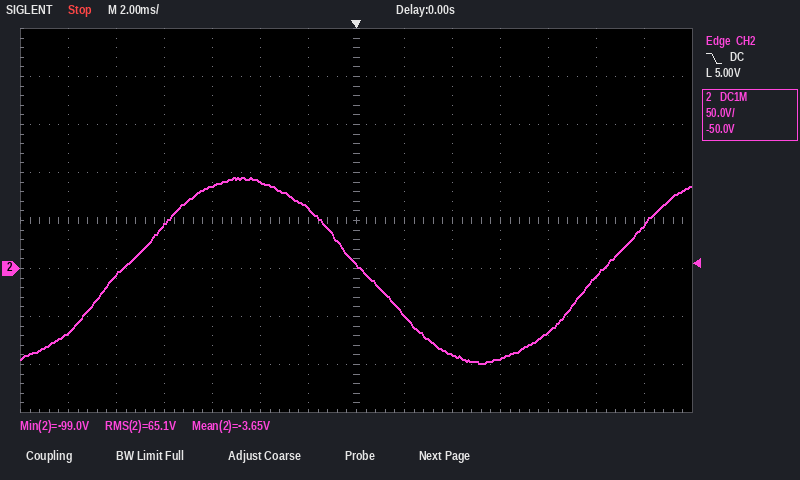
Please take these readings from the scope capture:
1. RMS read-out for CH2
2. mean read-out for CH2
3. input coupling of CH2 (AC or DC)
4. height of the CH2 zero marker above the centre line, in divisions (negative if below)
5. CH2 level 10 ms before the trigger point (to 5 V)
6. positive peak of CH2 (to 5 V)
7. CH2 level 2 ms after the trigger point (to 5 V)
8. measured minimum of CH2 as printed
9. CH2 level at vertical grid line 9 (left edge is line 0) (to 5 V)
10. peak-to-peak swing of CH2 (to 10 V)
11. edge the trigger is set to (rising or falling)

65.1 V
-3.65 V
DC
-1.0 div
-5 V
95 V
-50 V
-99.0 V
-90 V
190 V
falling
